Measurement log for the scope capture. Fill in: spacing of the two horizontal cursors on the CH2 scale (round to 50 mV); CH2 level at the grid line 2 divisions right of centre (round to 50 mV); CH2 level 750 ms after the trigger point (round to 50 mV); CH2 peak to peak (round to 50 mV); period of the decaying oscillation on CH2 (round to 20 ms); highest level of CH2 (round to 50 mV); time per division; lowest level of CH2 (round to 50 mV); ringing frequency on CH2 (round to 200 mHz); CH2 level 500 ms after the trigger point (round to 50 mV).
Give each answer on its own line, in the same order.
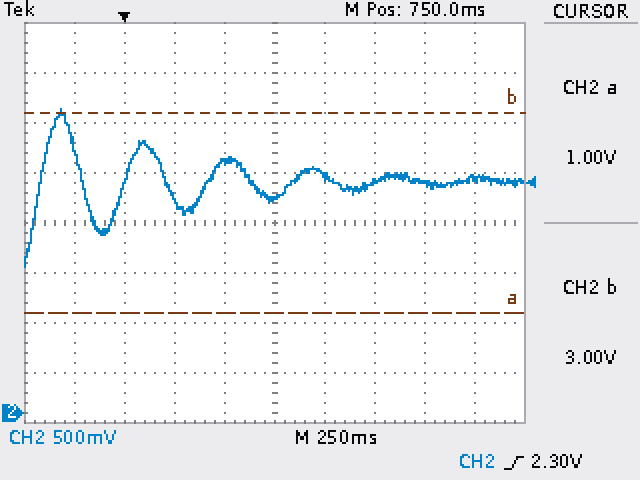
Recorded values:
2.00 V
2.30 V
2.15 V
1.60 V
420 ms
3.05 V
250 ms
1.45 V
2.4 Hz
2.50 V
